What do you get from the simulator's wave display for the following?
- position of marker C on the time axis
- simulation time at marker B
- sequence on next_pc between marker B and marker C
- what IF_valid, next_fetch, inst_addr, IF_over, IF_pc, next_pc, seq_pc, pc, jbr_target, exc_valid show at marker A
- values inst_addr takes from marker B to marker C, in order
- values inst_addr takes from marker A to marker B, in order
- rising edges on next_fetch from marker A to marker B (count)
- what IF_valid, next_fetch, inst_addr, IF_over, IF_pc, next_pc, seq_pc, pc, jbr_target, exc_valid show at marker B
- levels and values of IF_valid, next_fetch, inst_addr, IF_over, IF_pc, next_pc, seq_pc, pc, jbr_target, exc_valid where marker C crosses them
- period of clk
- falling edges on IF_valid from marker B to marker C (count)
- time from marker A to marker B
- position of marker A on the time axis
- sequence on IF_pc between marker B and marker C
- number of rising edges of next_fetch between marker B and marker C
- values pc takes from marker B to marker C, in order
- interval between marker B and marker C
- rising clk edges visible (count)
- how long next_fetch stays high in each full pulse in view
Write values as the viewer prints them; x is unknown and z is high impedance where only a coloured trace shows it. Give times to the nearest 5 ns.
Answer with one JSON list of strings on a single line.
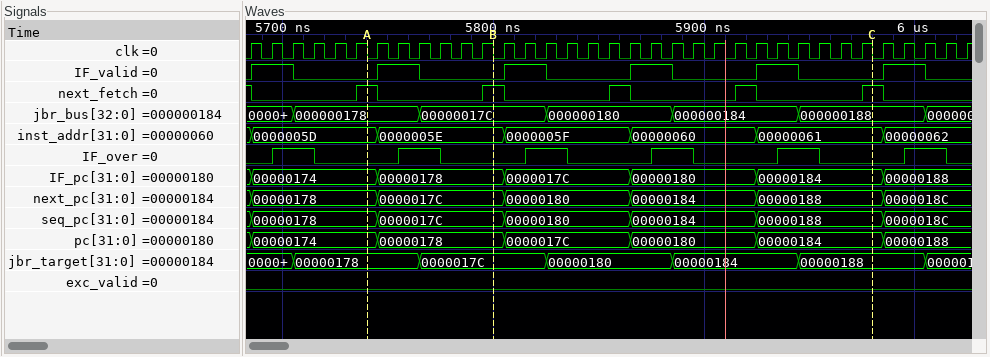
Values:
["5980 ns", "5800 ns", "0000017C, 00000180, 00000184, 00000188", "IF_valid=0, next_fetch=1, inst_addr=0000005D, IF_over=0, IF_pc=00000174, next_pc=00000178, seq_pc=00000178, pc=00000174, jbr_target=00000178, exc_valid=0", "0000005E, 0000005F, 00000060, 00000061", "0000005D, 0000005E", "1", "IF_valid=0, next_fetch=1, inst_addr=0000005E, IF_over=0, IF_pc=00000178, next_pc=0000017C, seq_pc=0000017C, pc=00000178, jbr_target=0000017C, exc_valid=0", "IF_valid=0, next_fetch=1, inst_addr=00000061, IF_over=0, IF_pc=00000184, next_pc=00000188, seq_pc=00000188, pc=00000184, jbr_target=00000188, exc_valid=0", "10 ns", "3", "60 ns", "5740 ns", "00000178, 0000017C, 00000180, 00000184", "3", "00000178, 0000017C, 00000180, 00000184", "180 ns", "35", "10 ns, 10 ns, 10 ns, 10 ns, 10 ns"]
